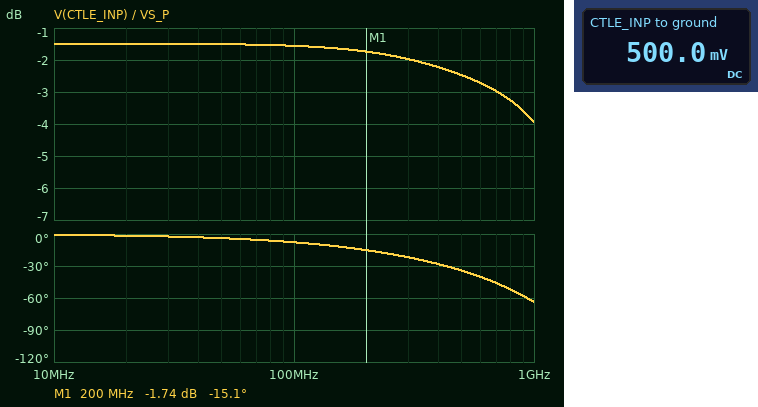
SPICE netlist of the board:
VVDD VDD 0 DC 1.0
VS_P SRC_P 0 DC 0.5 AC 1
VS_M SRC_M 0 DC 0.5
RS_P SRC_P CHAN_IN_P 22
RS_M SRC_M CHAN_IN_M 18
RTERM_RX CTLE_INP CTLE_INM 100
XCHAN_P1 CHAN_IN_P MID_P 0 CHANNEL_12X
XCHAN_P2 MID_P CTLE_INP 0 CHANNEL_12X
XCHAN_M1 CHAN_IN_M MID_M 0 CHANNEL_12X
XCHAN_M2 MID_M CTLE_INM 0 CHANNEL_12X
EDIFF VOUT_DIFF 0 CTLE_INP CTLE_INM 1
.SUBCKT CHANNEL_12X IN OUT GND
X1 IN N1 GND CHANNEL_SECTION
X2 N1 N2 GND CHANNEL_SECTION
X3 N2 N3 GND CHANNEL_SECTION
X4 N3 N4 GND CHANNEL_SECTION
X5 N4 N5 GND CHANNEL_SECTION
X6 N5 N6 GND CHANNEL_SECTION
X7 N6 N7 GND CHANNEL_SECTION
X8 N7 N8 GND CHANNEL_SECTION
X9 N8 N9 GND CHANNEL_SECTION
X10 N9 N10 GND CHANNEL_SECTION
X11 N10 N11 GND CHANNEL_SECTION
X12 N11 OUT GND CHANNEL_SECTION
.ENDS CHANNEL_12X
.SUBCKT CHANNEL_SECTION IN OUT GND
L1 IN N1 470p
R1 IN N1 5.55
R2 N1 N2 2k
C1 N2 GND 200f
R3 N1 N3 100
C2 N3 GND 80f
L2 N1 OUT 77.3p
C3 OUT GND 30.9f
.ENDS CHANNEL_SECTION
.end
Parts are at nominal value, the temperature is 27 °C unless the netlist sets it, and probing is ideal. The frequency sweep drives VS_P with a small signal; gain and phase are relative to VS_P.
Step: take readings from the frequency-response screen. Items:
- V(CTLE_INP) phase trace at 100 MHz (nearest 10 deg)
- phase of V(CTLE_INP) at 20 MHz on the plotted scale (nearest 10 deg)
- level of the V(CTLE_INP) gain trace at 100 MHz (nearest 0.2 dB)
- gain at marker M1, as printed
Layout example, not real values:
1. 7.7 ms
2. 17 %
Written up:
1. -10 deg
2. 0 deg
3. -1.6 dB
4. -1.74 dB
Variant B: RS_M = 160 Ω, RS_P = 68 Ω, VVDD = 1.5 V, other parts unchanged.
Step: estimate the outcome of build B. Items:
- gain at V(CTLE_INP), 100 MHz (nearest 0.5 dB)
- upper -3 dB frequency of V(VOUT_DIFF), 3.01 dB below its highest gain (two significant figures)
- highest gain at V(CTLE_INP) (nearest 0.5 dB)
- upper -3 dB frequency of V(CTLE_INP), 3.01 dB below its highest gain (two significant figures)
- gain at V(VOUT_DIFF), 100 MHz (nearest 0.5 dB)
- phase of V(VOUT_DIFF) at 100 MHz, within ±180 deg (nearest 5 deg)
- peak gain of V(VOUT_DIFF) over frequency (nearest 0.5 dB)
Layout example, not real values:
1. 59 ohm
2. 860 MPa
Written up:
1. -3.0 dB
2. 1.0 GHz
3. -2.0 dB
4. 280 MHz
5. -9.5 dB
6. 0 deg
7. -9.0 dB
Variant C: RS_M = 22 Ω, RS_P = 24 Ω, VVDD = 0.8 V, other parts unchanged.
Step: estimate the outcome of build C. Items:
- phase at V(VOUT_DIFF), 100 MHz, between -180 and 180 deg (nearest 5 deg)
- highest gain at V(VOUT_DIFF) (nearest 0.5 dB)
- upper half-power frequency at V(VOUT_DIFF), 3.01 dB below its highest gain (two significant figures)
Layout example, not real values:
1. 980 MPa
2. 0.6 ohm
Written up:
1. -10 deg
2. -3.5 dB
3. 600 MHz
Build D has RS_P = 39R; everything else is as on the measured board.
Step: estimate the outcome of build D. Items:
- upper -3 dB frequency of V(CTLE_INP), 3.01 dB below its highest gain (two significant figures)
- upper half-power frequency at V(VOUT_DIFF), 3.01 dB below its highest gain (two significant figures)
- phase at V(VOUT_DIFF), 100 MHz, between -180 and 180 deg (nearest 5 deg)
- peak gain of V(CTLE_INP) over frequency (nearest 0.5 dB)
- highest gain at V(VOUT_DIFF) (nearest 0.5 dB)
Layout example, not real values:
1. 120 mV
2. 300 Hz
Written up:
1. 890 MHz
2. 480 MHz
3. -15 deg
4. -2.5 dB
5. -4.0 dB
